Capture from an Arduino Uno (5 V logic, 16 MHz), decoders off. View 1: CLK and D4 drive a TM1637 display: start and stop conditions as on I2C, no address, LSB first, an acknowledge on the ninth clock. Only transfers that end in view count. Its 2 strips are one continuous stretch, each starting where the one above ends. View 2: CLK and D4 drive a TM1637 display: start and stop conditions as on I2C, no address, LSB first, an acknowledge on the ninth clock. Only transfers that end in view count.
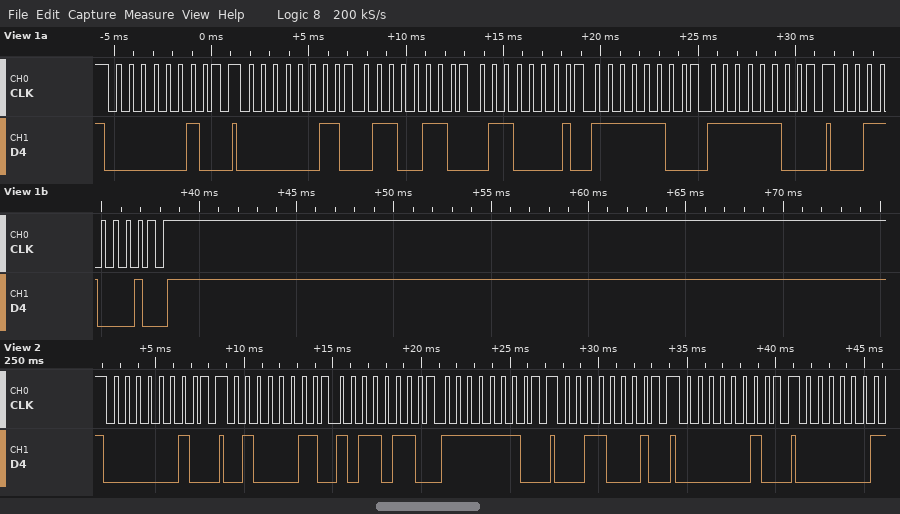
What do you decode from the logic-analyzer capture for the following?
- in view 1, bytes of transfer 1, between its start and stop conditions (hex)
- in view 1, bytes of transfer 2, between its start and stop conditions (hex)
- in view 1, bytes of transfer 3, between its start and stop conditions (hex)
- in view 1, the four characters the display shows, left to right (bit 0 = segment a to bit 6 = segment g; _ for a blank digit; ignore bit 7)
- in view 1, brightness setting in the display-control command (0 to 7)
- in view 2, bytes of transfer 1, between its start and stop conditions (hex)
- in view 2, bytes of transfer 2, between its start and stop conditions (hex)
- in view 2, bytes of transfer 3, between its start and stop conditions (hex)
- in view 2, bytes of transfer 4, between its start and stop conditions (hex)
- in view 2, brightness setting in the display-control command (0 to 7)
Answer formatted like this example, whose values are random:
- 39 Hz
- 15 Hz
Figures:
- 40
- C0 66 86 3F 3F
- 8C
- 4100
- 4
- 40
- C2 6D 7F
- 8C
- 40
- 4
